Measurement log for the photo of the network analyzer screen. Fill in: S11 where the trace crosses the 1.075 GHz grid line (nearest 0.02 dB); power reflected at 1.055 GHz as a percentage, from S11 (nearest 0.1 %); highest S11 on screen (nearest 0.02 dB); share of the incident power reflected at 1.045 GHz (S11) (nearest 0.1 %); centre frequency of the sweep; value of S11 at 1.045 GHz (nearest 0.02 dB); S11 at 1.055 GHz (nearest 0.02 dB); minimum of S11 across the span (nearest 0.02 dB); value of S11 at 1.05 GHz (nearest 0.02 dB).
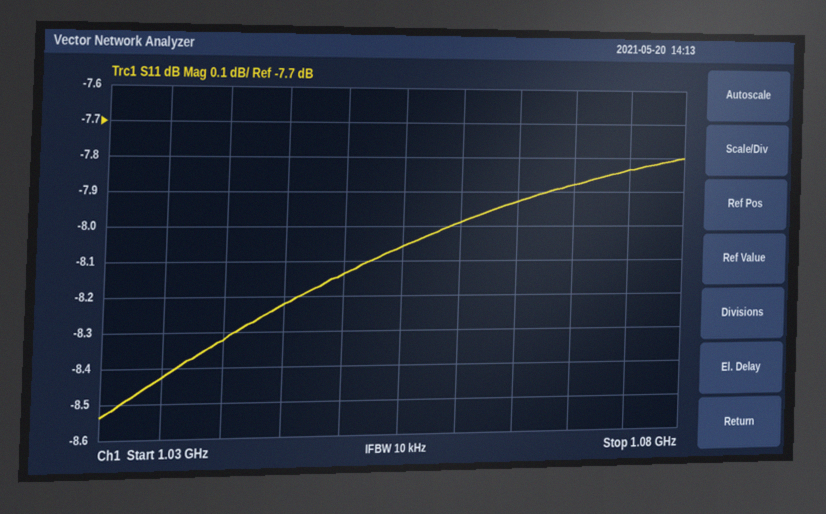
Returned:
-7.84 dB
15.6 %
-7.80 dB
15.1 %
1.055 GHz
-8.22 dB
-8.06 dB
-8.54 dB
-8.14 dB
